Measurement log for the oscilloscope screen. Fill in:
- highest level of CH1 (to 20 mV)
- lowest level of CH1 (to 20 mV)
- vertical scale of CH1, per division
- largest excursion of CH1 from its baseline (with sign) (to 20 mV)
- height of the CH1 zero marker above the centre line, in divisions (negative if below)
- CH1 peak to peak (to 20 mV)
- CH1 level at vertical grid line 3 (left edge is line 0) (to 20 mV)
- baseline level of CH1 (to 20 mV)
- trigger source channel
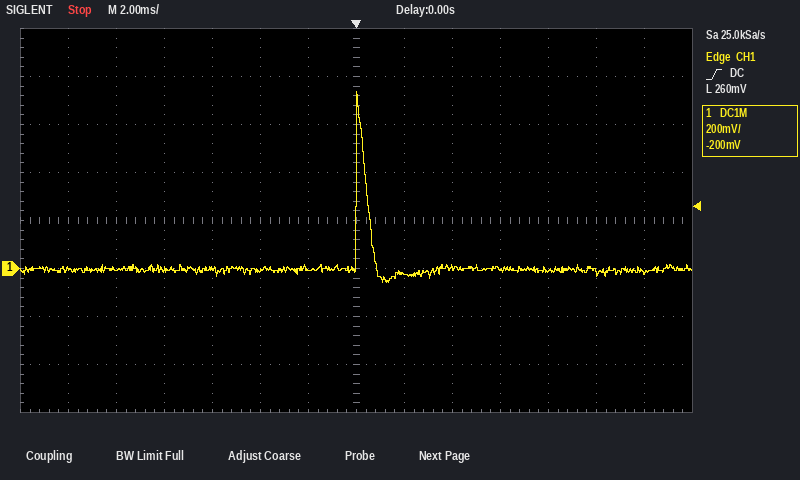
740 mV
-60 mV
200 mV
+740 mV
-1.0 div
800 mV
0 mV
0 mV
CH1
